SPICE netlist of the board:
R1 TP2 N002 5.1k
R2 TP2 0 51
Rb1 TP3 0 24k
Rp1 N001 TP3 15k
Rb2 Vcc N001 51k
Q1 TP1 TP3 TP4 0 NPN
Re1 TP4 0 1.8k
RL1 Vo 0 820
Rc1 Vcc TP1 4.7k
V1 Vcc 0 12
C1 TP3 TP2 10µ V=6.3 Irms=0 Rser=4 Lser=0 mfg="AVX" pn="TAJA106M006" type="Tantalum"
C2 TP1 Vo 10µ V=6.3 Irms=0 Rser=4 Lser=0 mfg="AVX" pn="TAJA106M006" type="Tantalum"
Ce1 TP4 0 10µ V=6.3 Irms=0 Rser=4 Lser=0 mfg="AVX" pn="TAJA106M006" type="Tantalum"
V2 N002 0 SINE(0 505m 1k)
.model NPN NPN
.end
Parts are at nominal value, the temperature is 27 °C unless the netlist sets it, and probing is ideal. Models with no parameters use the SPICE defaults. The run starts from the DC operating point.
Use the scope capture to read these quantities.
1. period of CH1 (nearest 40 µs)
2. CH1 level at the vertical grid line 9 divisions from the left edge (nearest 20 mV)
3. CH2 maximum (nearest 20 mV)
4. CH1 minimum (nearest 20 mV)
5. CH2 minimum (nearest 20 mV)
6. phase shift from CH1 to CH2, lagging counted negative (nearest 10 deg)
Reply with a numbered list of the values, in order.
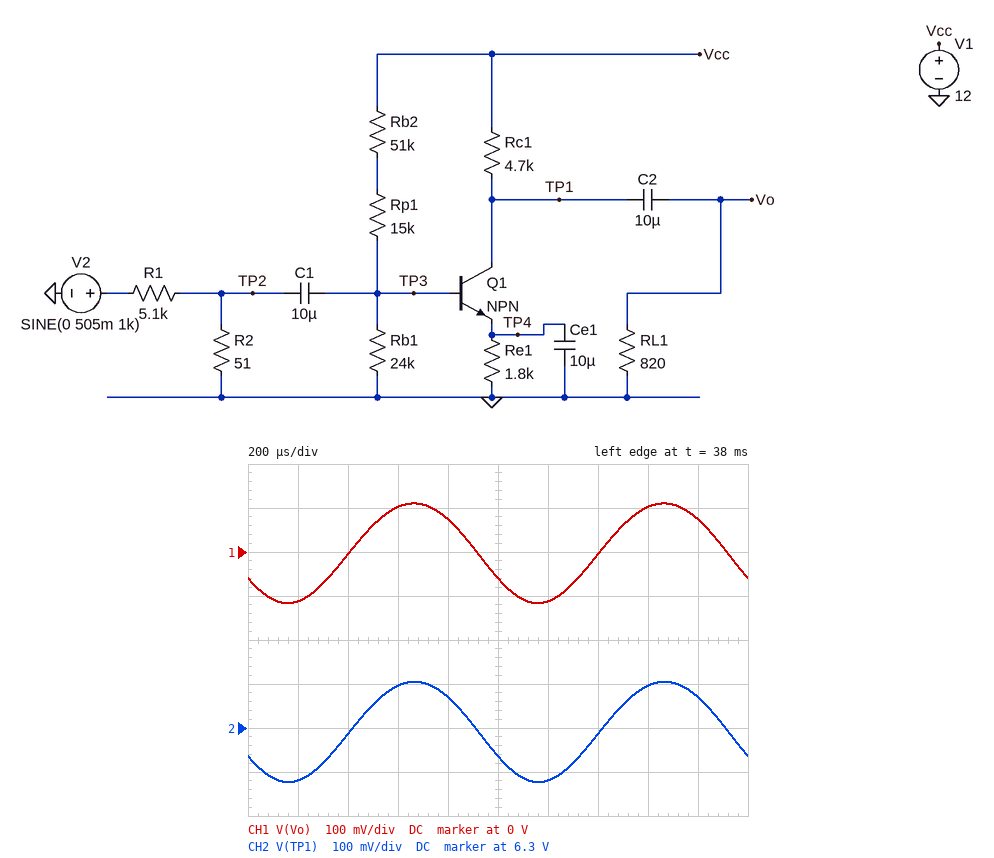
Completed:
1. 1.00 ms
2. 80 mV
3. 6.40 V
4. -120 mV
5. 6.18 V
6. 0 deg
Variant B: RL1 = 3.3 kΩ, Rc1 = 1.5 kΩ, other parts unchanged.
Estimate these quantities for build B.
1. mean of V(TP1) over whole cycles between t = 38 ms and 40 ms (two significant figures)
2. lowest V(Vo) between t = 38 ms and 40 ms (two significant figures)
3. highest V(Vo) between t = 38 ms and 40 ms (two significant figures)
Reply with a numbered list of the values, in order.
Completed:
1. 10 V
2. -170 mV
3. 160 mV
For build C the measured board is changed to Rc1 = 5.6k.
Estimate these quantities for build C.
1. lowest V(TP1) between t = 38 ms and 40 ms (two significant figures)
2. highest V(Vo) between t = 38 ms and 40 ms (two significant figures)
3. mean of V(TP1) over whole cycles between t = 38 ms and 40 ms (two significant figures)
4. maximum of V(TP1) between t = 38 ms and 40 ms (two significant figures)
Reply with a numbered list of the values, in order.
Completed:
1. 5.1 V
2. 110 mV
3. 5.2 V
4. 5.3 V
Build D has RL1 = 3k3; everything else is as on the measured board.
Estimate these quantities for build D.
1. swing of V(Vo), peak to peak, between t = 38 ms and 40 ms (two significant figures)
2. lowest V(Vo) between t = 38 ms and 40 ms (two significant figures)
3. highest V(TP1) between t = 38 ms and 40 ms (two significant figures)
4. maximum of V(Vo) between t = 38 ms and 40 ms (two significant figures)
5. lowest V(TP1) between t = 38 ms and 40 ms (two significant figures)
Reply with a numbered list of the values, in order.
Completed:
1. 630 mV
2. -320 mV
3. 6.6 V
4. 310 mV
5. 6.0 V
